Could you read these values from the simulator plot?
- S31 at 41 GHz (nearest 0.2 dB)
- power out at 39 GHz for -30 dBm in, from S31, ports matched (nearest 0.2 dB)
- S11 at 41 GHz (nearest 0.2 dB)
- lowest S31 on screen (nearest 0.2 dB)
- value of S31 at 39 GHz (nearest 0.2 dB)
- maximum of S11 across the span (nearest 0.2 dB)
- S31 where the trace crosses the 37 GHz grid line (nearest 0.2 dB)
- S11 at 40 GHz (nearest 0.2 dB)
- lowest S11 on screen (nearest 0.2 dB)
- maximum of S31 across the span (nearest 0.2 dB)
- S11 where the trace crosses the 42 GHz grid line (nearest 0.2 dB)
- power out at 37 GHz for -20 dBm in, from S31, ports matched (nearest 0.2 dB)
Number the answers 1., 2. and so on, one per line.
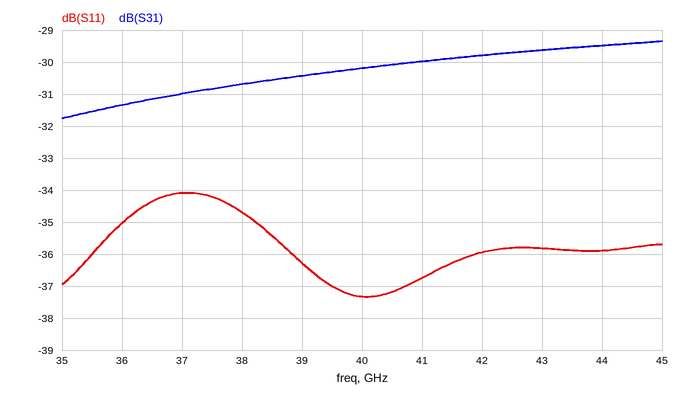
1. -30.0 dB
2. -60.4 dBm
3. -36.8 dB
4. -31.8 dB
5. -30.4 dB
6. -34.0 dB
7. -31.0 dB
8. -37.4 dB
9. -37.4 dB
10. -29.4 dB
11. -36.0 dB
12. -51.0 dBm
